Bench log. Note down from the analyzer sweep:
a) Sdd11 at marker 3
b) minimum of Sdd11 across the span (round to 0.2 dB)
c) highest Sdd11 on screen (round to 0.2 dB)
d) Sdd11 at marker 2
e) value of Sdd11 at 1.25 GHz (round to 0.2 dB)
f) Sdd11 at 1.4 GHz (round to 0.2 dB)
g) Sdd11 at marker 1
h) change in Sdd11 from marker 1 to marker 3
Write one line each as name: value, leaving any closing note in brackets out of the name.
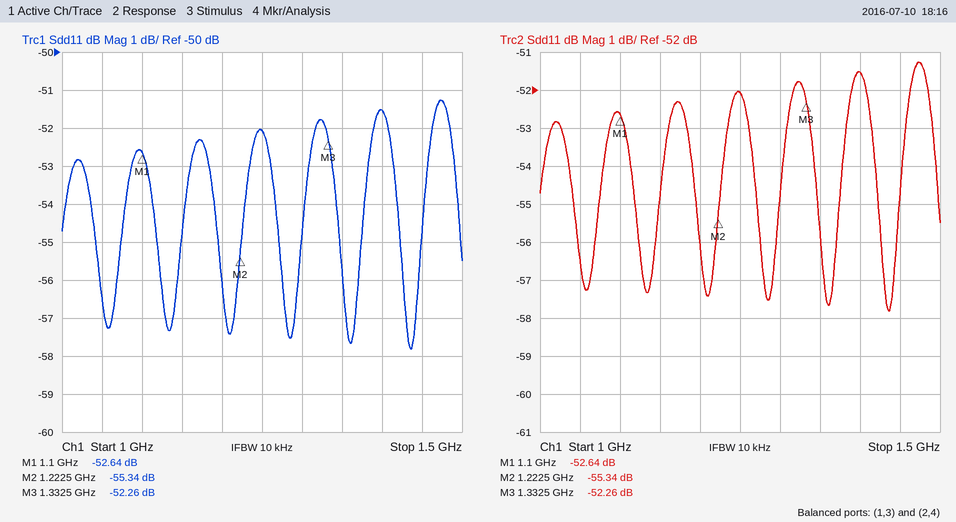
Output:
Sdd11 at marker 3: -52.26 dB
minimum of Sdd11 across the span: -57.8 dB
highest Sdd11 on screen: -51.2 dB
Sdd11 at marker 2: -55.34 dB
value of Sdd11 at 1.25 GHz: -52.0 dB
Sdd11 at 1.4 GHz: -51.6 dB
Sdd11 at marker 1: -52.64 dB
change in Sdd11 from marker 1 to marker 3: 0.38 dB
